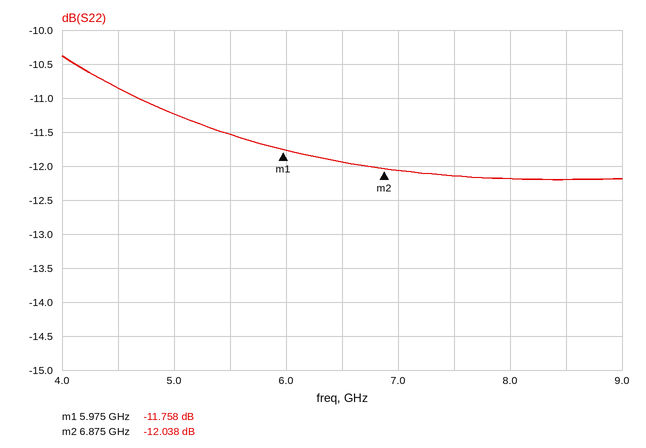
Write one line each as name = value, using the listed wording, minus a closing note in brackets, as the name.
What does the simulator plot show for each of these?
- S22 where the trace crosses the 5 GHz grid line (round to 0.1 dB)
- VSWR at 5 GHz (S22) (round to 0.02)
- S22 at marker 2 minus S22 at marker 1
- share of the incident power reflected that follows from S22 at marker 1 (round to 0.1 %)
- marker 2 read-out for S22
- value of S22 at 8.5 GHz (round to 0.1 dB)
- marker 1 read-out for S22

S22 where the trace crosses the 5 GHz grid line = -11.2 dB
VSWR at 5 GHz (S22) = 1.76
S22 at marker 2 minus S22 at marker 1 = -0.280 dB
share of the incident power reflected that follows from S22 at marker 1 = 6.7 %
marker 2 read-out for S22 = -12.038 dB
value of S22 at 8.5 GHz = -12.2 dB
marker 1 read-out for S22 = -11.758 dB
